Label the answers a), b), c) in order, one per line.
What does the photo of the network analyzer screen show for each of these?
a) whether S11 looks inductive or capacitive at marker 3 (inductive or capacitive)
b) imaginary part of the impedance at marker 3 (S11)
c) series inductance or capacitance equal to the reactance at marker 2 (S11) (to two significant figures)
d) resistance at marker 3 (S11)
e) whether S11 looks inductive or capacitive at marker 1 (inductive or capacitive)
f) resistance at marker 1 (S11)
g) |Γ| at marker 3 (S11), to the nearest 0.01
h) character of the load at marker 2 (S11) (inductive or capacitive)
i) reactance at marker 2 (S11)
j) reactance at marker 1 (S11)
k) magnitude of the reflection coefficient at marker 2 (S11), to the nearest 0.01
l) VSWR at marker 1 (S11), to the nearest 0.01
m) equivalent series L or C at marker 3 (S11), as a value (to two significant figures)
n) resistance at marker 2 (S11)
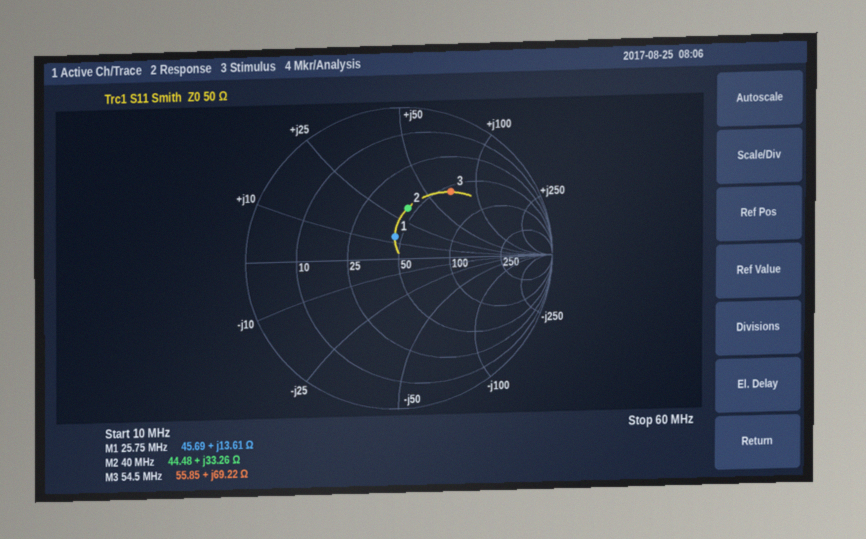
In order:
a) inductive
b) +69.22 Ω
c) 130 nH
d) 55.85 Ω
e) inductive
f) 45.69 Ω
g) 0.55
h) inductive
i) +33.26 Ω
j) +13.61 Ω
k) 0.34
l) 1.35
m) 200 nH
n) 44.48 Ω
